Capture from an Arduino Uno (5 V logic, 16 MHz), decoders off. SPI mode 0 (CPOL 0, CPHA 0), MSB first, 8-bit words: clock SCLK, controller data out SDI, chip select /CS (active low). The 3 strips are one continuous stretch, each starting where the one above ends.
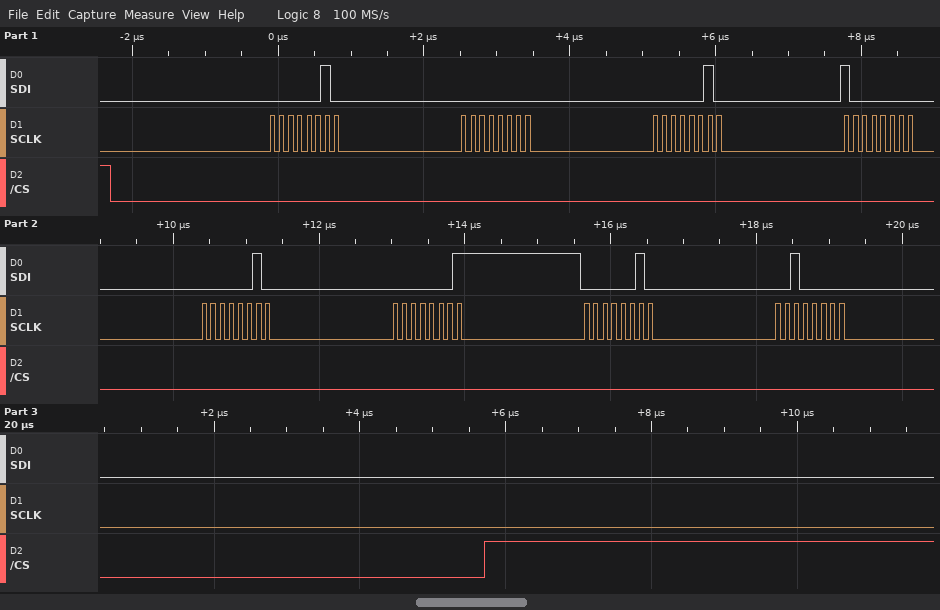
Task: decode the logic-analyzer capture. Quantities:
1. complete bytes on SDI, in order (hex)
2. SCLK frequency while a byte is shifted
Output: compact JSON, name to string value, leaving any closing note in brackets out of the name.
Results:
{"complete bytes on SDI, in order": "02 00 02 80 02 01 02 20", "SCLK frequency while a byte is shifted": "8 MHz"}
